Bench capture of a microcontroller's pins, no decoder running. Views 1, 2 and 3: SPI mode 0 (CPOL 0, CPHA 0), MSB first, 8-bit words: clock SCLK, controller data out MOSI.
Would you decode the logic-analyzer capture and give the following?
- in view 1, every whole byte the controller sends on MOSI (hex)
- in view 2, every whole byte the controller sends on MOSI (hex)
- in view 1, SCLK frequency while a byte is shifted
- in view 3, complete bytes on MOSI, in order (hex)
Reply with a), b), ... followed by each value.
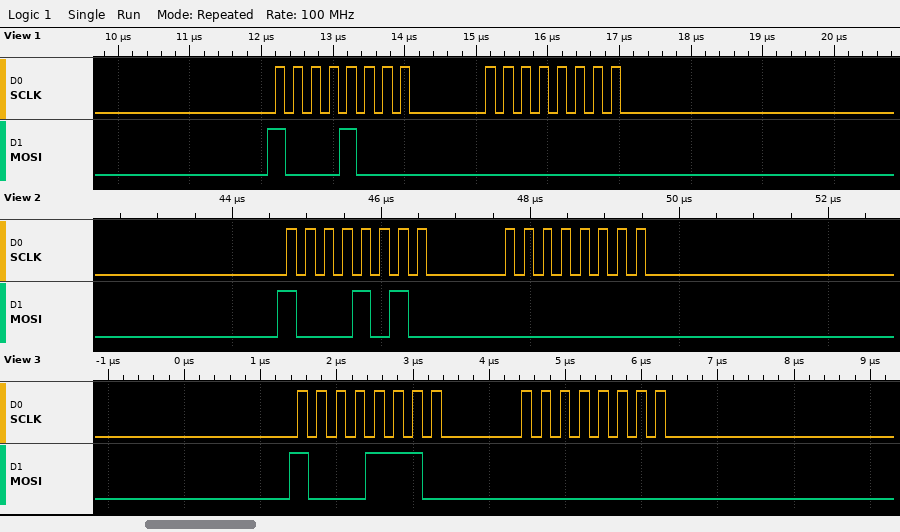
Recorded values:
a) 88 00
b) 0x8A 0x00
c) 4 MHz
d) 0x8E 0x00
